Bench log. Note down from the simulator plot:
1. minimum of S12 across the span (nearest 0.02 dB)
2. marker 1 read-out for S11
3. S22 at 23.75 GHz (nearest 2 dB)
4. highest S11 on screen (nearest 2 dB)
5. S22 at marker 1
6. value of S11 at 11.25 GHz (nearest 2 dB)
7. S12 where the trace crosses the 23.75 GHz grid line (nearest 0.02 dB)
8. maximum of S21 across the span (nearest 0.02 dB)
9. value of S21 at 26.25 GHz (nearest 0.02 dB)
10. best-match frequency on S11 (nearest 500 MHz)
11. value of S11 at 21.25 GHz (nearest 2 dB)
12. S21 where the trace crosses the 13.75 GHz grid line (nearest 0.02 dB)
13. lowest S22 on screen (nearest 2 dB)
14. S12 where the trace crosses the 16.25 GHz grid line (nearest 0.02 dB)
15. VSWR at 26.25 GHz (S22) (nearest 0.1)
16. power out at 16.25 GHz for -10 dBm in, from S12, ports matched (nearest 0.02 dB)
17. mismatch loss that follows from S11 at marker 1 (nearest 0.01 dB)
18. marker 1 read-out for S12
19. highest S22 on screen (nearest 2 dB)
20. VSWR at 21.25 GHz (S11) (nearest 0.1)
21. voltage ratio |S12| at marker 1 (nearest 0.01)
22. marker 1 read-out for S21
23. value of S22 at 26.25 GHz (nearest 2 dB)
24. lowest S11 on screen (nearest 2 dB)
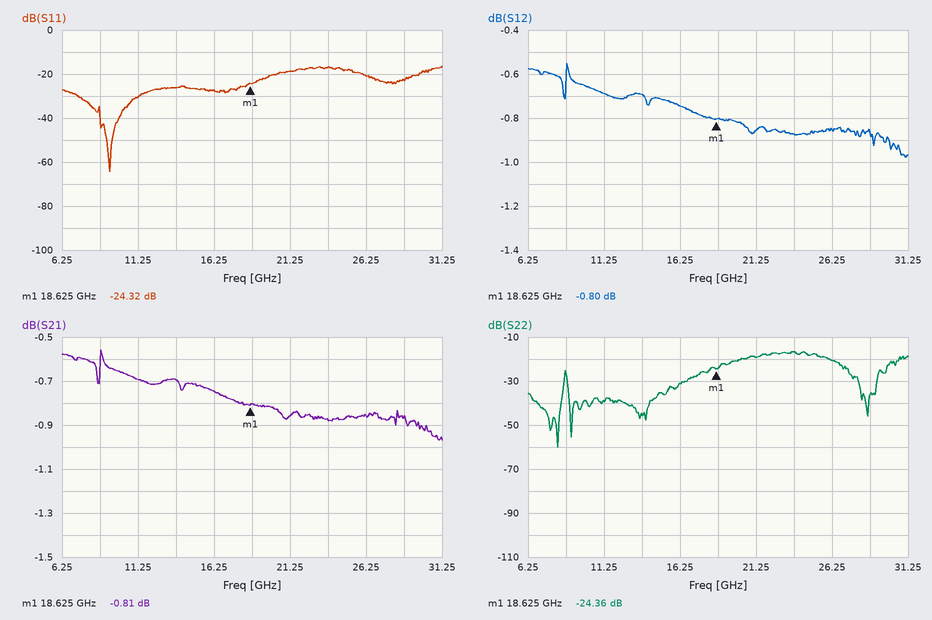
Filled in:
-0.98 dB
-24.32 dB
-16 dB
-16 dB
-24.36 dB
-30 dB
-0.88 dB
-0.56 dB
-0.86 dB
9.5 GHz
-18 dB
-0.70 dB
-60 dB
-0.74 dB
1.2
-10.74 dBm
0.02 dB
-0.80 dB
-16 dB
1.3
0.91
-0.81 dB
-20 dB
-64 dB
